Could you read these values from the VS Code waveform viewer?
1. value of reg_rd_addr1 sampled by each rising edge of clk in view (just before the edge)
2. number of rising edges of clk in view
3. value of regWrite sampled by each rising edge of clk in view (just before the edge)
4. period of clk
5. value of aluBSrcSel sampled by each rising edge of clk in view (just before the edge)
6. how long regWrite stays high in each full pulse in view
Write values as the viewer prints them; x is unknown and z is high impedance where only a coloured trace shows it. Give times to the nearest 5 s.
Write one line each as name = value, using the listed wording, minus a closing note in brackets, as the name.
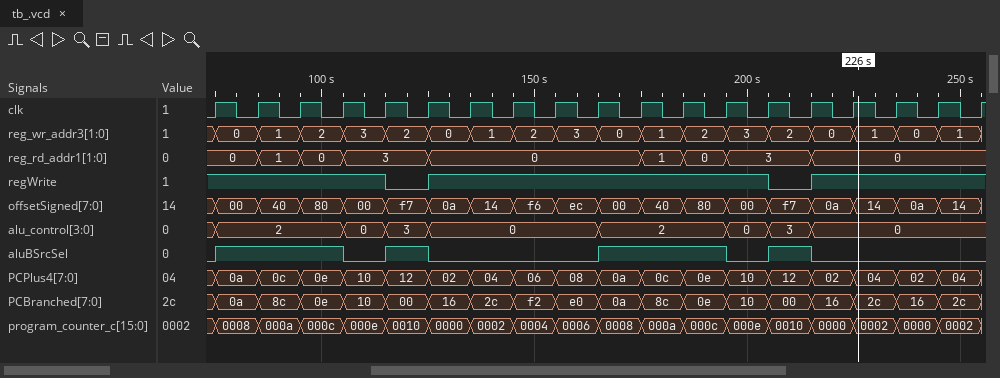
value of reg_rd_addr1 sampled by each rising edge of clk in view = 0, 0, 1, 0, 3, 3, 0, 0, 0, 0, 0, 1, 0, 3, 3, 0, 0, 0, 0
number of rising edges of clk in view = 19
value of regWrite sampled by each rising edge of clk in view = 1 1 1 1 1 0 1 1 1 1 1 1 1 1 0 1 1 1 1
period of clk = 10 s
value of aluBSrcSel sampled by each rising edge of clk in view = 0 1 1 1 0 1 0 0 0 0 1 1 1 0 1 0 0 0 0
how long regWrite stays high in each full pulse in view = 80 s
